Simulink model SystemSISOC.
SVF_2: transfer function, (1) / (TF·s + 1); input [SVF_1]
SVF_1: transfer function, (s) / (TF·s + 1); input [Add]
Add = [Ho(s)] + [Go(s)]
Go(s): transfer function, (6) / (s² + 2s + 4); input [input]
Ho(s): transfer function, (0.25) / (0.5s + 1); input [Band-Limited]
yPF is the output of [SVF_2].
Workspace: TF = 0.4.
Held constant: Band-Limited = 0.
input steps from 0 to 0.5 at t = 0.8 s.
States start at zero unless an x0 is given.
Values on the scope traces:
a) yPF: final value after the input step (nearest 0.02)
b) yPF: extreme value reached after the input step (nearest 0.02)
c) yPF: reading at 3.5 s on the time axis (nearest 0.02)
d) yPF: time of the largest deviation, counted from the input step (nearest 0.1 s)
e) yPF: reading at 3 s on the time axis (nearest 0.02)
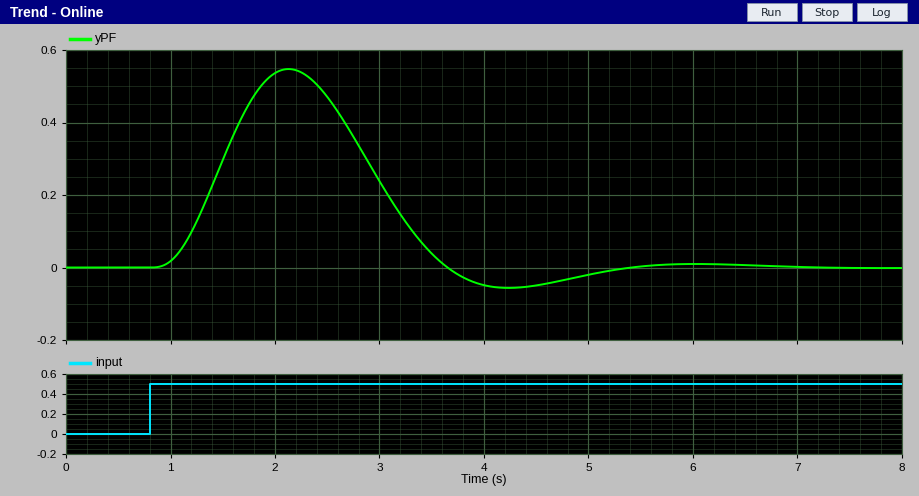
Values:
0.00
0.54
0.04
1.3 s
0.24
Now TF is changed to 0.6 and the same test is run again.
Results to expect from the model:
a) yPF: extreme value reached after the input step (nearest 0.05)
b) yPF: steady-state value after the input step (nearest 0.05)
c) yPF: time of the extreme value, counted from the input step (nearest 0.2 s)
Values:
0.45
0.00
1.6 s
